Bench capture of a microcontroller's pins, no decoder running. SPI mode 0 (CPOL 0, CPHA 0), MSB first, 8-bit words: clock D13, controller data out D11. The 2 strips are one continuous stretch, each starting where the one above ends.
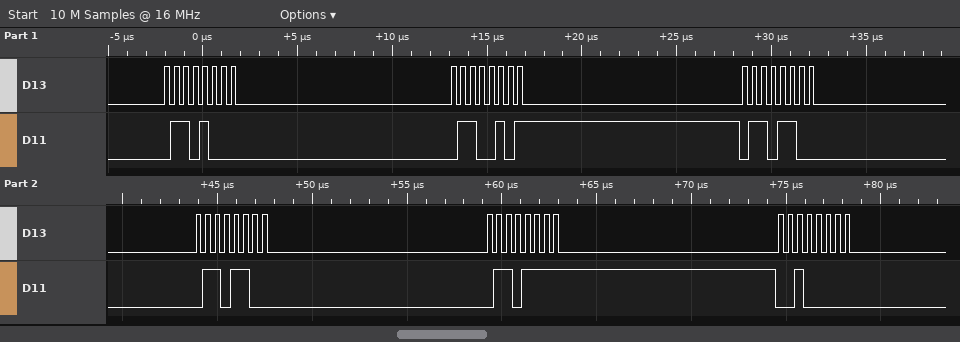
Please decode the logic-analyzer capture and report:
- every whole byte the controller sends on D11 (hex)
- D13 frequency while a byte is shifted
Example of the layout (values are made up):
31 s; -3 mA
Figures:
68 65 6C 6C 6F 20; 2 MHz
